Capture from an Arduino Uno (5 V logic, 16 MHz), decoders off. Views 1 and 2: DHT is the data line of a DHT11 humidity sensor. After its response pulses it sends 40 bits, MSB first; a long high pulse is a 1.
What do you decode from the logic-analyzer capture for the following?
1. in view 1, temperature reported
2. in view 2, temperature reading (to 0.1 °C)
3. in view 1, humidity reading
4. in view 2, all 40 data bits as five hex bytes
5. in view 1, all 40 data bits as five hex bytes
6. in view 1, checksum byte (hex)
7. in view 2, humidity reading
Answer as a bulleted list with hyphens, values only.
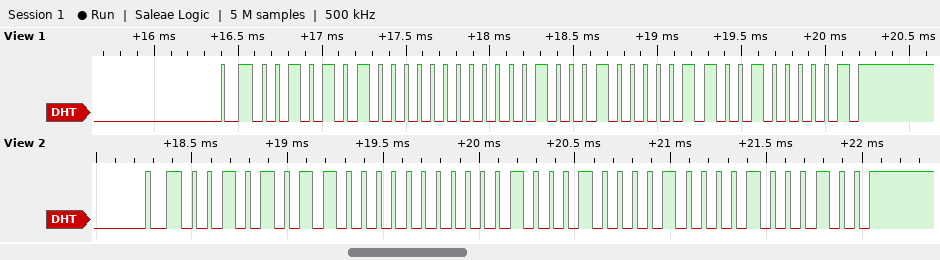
- 17.6 °C
- 17.8 °C
- 42 %
- 2B 00 11 08 44
- 2A 00 11 06 41
- 0x41
- 43 %
